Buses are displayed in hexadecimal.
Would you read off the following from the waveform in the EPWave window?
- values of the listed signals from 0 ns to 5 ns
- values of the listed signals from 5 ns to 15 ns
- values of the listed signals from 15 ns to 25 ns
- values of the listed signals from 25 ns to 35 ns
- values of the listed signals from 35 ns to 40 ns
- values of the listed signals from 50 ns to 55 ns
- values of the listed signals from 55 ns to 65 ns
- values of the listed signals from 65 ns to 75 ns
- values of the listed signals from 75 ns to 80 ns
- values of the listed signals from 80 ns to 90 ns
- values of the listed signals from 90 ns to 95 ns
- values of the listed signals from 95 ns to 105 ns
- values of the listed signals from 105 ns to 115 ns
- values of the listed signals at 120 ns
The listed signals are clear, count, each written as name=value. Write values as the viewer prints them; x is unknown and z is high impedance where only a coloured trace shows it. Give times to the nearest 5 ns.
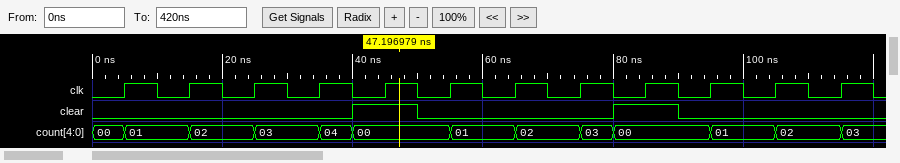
clear=0, count=00
clear=0, count=01
clear=0, count=02
clear=0, count=03
clear=0, count=04
clear=0, count=00
clear=0, count=01
clear=0, count=02
clear=0, count=03
clear=1, count=00
clear=0, count=00
clear=0, count=01
clear=0, count=02
clear=0, count=03
